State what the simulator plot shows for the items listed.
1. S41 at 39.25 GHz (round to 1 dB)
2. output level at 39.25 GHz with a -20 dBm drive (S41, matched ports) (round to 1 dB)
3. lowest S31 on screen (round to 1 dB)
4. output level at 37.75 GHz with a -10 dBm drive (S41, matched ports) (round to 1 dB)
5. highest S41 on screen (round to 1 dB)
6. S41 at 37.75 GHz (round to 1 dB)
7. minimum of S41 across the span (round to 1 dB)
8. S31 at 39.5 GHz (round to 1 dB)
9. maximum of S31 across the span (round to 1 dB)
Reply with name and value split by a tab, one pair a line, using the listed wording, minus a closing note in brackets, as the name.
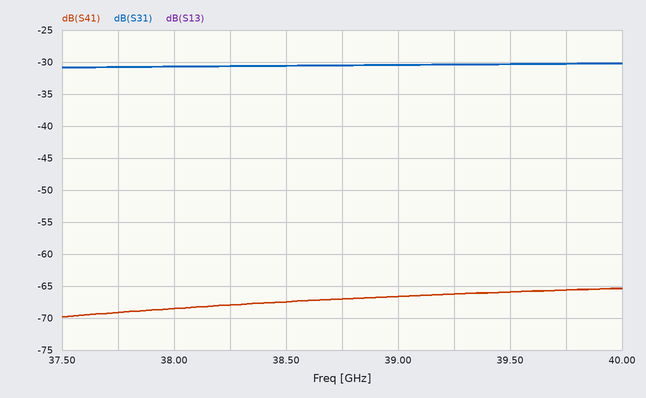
S41 at 39.25 GHz	-66 dB
output level at 39.25 GHz with a -20 dBm drive (S41, matched ports)	-86 dBm
lowest S31 on screen	-31 dB
output level at 37.75 GHz with a -10 dBm drive (S41, matched ports)	-79 dBm
highest S41 on screen	-65 dB
S41 at 37.75 GHz	-69 dB
minimum of S41 across the span	-70 dB
S31 at 39.5 GHz	-30 dB
maximum of S31 across the span	-30 dB
